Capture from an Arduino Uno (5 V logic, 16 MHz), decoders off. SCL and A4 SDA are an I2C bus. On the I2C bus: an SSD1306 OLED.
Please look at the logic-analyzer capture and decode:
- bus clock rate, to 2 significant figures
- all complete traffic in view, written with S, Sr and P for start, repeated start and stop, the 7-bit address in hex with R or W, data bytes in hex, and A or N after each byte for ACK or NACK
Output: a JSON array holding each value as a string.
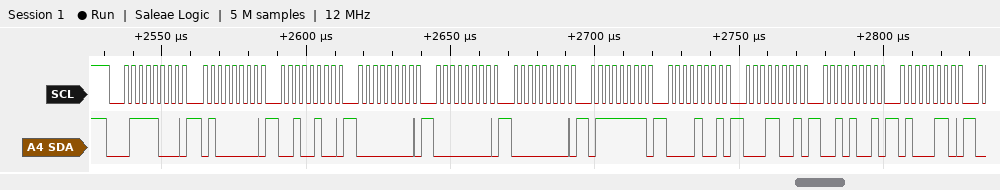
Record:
["400 kHz", "S 3CW A 40 A 24 A 00 A 00 A 00 A 7F A 09 A 19 A 29 A 46 A"]
